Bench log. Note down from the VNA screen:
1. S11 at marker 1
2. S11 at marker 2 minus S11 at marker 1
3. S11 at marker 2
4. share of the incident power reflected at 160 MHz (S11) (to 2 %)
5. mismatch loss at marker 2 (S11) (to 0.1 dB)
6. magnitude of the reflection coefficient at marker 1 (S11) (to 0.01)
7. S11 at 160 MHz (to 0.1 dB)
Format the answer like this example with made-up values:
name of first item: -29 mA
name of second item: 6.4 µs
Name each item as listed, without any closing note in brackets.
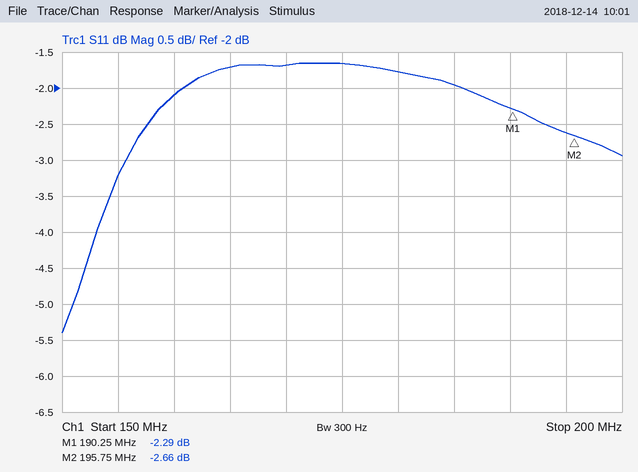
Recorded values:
S11 at marker 1: -2.29 dB
S11 at marker 2 minus S11 at marker 1: -0.37 dB
S11 at marker 2: -2.66 dB
share of the incident power reflected at 160 MHz (S11): 62 %
mismatch loss at marker 2 (S11): 3.4 dB
magnitude of the reflection coefficient at marker 1 (S11): 0.77
S11 at 160 MHz: -2.1 dB
